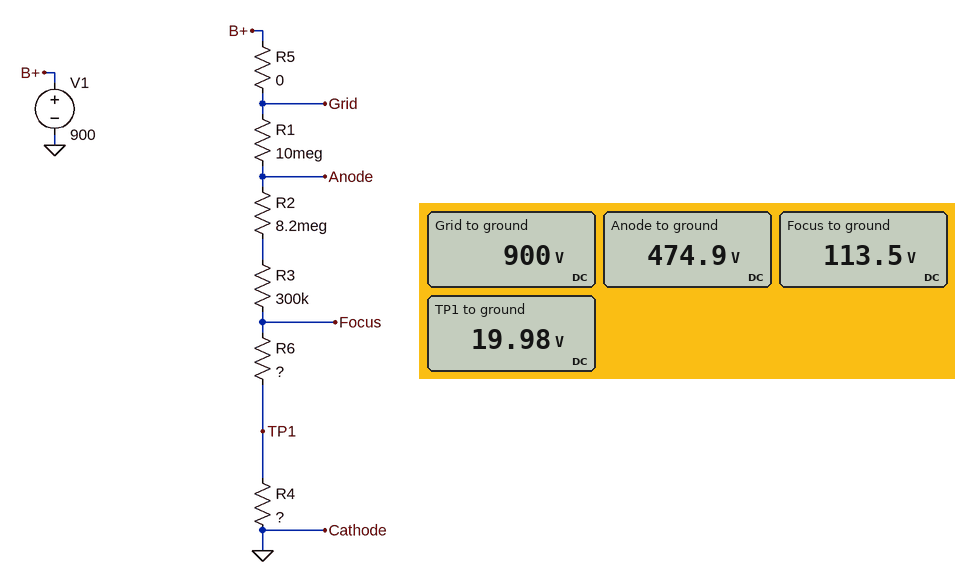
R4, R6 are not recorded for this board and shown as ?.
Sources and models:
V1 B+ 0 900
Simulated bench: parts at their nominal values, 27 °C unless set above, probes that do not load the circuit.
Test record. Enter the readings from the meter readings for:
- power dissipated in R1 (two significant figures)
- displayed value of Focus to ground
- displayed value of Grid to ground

18 mW
113.5 V
900 V
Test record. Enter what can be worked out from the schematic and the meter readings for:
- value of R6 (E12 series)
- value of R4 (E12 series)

2.2 MΩ
470 kΩ
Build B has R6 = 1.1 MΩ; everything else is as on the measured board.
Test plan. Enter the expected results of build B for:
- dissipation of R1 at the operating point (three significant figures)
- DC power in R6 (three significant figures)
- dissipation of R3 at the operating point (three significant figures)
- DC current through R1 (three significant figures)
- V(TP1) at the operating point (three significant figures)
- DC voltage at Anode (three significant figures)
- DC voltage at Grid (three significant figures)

20.1 mW
2.21 mW
603 µW
44.8 µA
21.1 V
452 V
900 V
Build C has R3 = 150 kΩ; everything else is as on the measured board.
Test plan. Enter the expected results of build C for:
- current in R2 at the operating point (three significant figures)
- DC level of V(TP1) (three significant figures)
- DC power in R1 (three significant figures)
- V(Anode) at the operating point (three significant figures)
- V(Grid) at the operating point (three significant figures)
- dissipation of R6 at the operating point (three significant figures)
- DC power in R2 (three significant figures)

42.8 µA
20.1 V
18.3 mW
472 V
900 V
4.03 mW
15.0 mW
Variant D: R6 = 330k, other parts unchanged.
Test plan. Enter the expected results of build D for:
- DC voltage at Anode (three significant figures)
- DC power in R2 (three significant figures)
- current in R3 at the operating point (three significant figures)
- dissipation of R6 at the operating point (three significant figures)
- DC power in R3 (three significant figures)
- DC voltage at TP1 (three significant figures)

434 V
17.8 mW
46.6 µA
718 µW
652 µW
21.9 V
